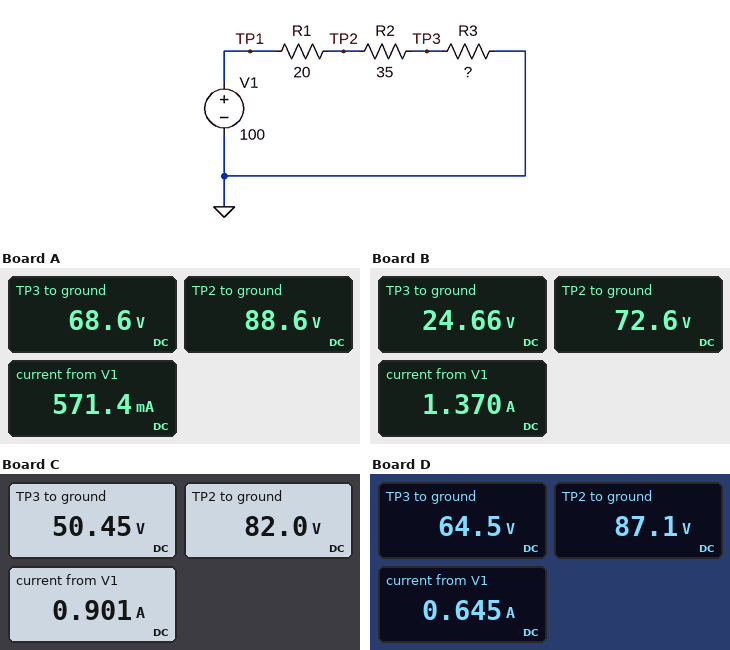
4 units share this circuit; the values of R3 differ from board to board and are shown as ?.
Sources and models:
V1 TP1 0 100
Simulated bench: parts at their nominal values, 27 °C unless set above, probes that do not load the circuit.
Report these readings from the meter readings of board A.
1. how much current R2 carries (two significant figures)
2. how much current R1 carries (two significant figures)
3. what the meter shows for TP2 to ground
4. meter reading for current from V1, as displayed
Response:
570 mA
570 mA
88.6 V
571.4 mA
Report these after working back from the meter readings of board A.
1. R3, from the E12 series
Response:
120 Ω
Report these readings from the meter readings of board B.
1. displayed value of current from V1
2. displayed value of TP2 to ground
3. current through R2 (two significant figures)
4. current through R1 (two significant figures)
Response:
1.370 A
72.6 V
1.4 A
1.4 A
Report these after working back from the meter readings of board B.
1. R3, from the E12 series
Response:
18 Ω
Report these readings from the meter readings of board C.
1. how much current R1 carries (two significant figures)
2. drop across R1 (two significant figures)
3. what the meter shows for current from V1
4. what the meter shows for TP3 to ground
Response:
900 mA
18 V
0.901 A
50.45 V
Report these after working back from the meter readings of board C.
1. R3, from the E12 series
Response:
56 Ω
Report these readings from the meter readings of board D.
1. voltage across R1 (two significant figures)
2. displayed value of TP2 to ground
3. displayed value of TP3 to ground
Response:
13 V
87.1 V
64.5 V
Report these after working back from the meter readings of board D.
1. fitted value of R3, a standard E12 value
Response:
100 Ω
